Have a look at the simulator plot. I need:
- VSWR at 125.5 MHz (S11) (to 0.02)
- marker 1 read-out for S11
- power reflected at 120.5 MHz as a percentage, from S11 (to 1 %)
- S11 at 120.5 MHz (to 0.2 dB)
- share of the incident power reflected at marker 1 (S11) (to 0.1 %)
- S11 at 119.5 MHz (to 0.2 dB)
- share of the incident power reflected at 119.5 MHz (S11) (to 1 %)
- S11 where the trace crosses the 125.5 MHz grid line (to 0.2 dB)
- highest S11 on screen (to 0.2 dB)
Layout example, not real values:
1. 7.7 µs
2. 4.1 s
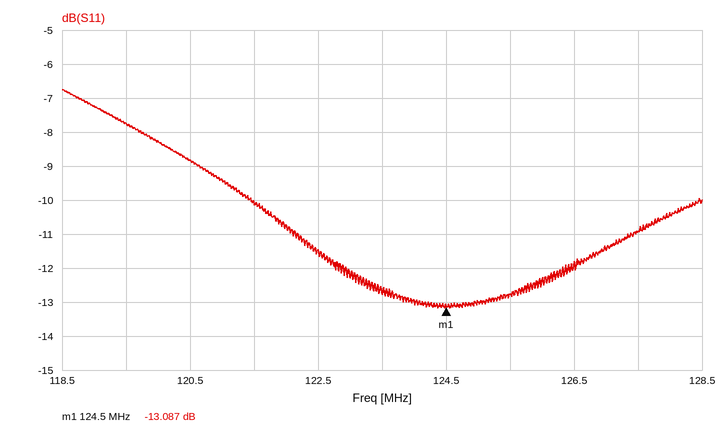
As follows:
1. 1.60
2. -13.087 dB
3. 13 %
4. -8.8 dB
5. 4.9 %
6. -7.8 dB
7. 17 %
8. -12.8 dB
9. -6.8 dB
